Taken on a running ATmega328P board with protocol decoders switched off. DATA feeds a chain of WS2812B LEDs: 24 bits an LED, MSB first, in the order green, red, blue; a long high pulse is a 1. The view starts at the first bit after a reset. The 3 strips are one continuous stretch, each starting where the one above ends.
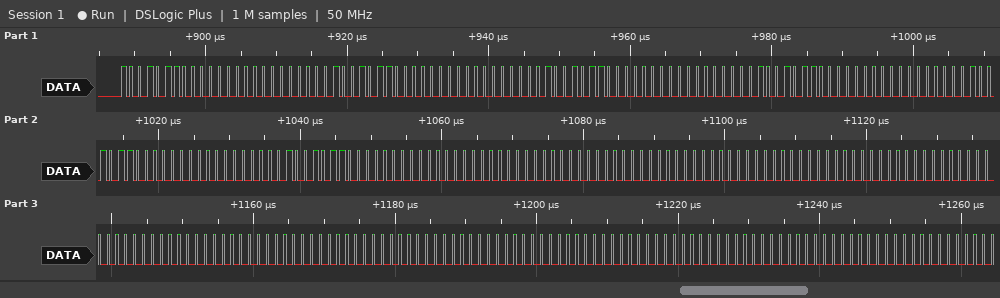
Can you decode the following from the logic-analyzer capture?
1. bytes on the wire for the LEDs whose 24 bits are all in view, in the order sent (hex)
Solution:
96 00 00 96 00 00 96 00 00 96 00 00 96 00 00 96 00 00 00 00 00 00 00 00 00 00 00 00 00 00 00 00 00 00 00 00
